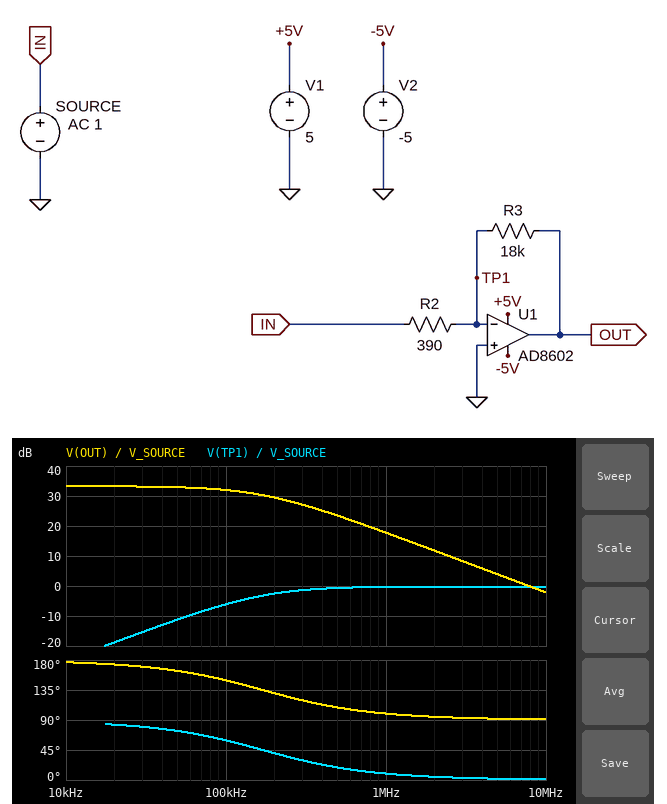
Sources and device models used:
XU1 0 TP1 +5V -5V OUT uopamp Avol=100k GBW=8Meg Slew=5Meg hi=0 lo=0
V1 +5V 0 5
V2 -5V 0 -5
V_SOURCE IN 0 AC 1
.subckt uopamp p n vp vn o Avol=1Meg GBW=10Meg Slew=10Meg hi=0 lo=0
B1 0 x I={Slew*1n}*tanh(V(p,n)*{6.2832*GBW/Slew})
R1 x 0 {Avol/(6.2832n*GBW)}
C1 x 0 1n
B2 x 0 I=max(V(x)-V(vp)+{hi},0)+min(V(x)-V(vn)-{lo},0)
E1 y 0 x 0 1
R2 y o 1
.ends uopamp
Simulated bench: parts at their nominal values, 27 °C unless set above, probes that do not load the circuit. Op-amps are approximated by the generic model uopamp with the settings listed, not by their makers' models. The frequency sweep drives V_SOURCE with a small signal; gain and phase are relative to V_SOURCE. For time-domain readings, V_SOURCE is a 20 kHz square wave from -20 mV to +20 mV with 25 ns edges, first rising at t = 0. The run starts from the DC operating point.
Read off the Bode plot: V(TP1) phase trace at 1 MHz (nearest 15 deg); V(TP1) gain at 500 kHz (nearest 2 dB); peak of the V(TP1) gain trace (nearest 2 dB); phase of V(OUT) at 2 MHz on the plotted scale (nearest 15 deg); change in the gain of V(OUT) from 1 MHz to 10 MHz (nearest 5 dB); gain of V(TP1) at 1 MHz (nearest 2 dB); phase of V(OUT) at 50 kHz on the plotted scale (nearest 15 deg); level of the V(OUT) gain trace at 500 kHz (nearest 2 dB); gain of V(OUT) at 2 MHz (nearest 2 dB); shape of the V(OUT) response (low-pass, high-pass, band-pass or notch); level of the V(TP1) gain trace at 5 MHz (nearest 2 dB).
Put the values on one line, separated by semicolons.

15 deg; 0 dB; 0 dB; 90 deg; -20 dB; 0 dB; 165 deg; 24 dB; 12 dB; low-pass; 0 dB
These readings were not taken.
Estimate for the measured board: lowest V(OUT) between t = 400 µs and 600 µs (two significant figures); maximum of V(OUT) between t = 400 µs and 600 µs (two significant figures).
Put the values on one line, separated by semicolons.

-920 mV; 920 mV
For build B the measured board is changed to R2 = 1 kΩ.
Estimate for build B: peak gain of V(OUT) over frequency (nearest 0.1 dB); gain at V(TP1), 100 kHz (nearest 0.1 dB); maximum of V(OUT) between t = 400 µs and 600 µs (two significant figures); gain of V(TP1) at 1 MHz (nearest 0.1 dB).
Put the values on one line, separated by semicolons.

25.1 dB; -13.2 dB; 360 mV; -1.2 dB
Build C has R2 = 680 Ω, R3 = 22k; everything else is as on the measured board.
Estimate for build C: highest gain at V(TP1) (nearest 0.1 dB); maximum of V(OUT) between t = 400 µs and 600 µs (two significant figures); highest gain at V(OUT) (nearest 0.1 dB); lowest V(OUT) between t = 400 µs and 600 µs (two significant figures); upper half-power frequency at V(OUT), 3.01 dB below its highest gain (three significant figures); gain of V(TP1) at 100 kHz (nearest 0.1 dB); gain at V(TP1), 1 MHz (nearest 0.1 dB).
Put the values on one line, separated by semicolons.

-0.3 dB; 650 mV; 30.2 dB; -650 mV; 240 kHz; -8.6 dB; -0.5 dB
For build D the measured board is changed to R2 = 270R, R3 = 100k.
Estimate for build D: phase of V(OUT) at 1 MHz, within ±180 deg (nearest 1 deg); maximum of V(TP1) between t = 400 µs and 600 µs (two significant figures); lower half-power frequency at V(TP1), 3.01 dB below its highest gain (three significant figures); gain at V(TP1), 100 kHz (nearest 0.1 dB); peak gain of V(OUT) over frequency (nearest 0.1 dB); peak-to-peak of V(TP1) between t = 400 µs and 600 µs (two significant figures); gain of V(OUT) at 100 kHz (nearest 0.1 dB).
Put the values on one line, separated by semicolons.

91 deg; 33 mV; 21.6 kHz; -0.2 dB; 51.3 dB; 67 mV; 37.8 dB
